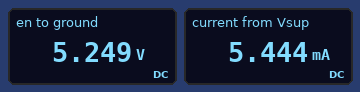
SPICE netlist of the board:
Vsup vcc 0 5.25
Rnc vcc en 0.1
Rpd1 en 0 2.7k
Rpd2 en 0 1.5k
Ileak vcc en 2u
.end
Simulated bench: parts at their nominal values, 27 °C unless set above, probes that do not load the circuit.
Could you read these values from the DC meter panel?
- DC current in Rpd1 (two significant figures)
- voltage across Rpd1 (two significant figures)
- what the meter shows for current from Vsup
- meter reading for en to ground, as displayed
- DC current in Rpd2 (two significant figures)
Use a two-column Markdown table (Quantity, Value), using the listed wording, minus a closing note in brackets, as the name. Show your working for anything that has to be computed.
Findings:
| Quantity | Value |
|---|---|
| DC current in Rpd1 | (5.249 V) / 2.7 kΩ = 1.9 mA |
| voltage across Rpd1 | 5.249 V = 5.2 V |
| what the meter shows for current from Vsup | 5.444 mA |
| meter reading for en to ground, as displayed | 5.249 V |
| DC current in Rpd2 | (5.249 V) / 1.5 kΩ = 3.5 mA |
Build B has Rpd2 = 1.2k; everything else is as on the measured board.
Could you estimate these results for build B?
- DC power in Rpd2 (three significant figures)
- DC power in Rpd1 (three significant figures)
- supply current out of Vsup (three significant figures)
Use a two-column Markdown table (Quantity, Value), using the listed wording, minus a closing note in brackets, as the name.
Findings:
| Quantity | Value |
|---|---|
| DC power in Rpd2 | 23.0 mW |
| DC power in Rpd1 | 10.2 mW |
| supply current out of Vsup | 6.32 mA |
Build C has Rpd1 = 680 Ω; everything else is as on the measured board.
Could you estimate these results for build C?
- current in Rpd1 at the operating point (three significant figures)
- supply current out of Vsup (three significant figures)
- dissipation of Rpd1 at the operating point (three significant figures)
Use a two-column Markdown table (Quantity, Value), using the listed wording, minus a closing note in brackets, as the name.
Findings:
| Quantity | Value |
|---|---|
| current in Rpd1 at the operating point | 7.72 mA |
| supply current out of Vsup | 11.2 mA |
| dissipation of Rpd1 at the operating point | 40.5 mW |
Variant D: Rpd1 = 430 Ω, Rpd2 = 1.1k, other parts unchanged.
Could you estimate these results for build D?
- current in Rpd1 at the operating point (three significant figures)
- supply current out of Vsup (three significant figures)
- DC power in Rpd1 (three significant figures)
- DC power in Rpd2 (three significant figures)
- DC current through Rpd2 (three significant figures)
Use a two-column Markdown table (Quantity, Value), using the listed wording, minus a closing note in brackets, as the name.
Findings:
| Quantity | Value |
|---|---|
| current in Rpd1 at the operating point | 12.2 mA |
| supply current out of Vsup | 17.0 mA |
| DC power in Rpd1 | 64.1 mW |
| DC power in Rpd2 | 25.0 mW |
| DC current through Rpd2 | 4.77 mA |
